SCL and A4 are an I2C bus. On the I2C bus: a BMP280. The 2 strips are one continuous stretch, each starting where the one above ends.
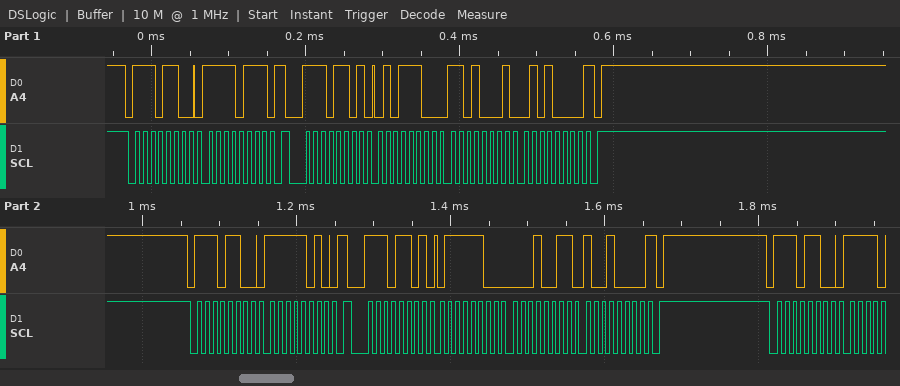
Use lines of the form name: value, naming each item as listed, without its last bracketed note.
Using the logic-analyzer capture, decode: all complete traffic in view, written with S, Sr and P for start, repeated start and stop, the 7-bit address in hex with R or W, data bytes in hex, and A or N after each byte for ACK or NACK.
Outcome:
all complete traffic in view, written with S, Sr and P for start, repeated start and stop, the 7-bit address in hex with R or W, data bytes in hex, and A or N after each byte for ACK or NACK: S 76W A F7 A Sr 76R A 5C A D1 A 50 N P S 76W A FA A Sr 76R A 7C A 13 A 90 N P S 76W A
